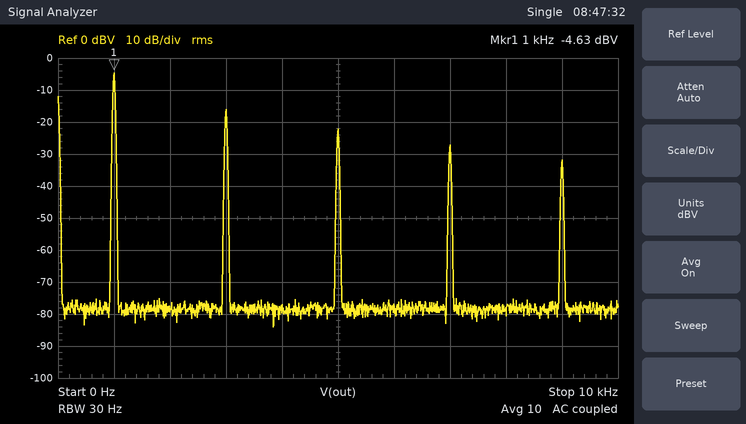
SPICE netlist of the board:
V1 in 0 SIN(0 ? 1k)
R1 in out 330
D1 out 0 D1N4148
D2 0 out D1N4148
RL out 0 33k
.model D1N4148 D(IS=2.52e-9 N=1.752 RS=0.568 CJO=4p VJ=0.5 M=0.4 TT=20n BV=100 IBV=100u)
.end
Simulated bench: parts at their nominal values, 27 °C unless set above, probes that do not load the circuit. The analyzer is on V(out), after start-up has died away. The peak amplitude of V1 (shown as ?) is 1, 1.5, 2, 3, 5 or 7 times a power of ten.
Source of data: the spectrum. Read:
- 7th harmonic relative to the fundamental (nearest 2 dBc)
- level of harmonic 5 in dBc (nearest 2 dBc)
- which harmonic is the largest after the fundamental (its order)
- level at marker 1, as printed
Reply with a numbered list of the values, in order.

1. -22 dBc
2. -18 dBc
3. 3
4. -4.63 dBV
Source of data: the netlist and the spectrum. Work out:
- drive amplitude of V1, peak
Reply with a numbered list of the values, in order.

1. 3 V
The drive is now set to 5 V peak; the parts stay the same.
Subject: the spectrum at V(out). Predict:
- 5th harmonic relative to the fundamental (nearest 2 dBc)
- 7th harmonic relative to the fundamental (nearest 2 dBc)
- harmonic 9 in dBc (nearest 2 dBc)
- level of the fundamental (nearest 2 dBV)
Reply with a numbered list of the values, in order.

1. -16 dBc
2. -20 dBc
3. -24 dBc
4. -4 dBV
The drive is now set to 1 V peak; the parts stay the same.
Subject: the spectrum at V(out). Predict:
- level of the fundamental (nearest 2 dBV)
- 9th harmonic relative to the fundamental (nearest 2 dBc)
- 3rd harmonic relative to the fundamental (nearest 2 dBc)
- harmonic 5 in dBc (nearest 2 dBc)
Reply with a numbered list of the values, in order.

1. -6 dBV
2. -42 dBc
3. -16 dBc
4. -34 dBc
